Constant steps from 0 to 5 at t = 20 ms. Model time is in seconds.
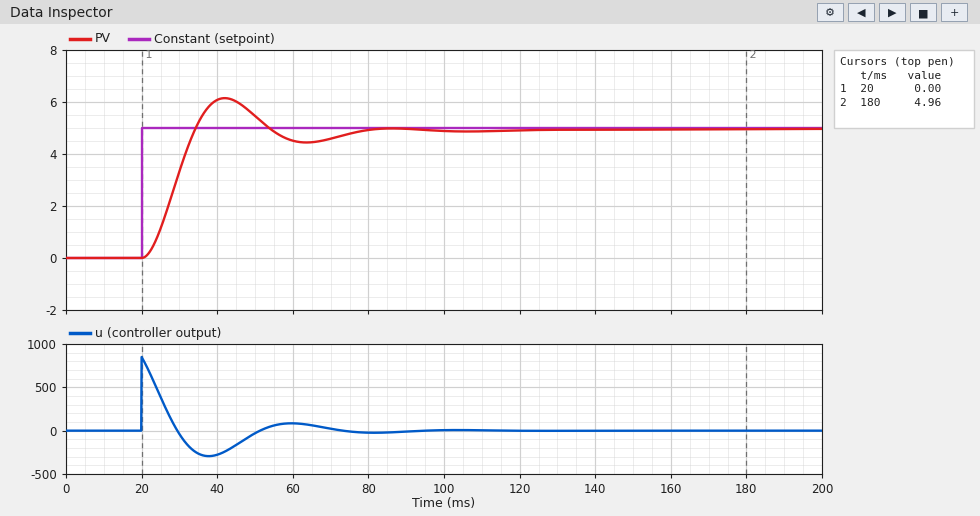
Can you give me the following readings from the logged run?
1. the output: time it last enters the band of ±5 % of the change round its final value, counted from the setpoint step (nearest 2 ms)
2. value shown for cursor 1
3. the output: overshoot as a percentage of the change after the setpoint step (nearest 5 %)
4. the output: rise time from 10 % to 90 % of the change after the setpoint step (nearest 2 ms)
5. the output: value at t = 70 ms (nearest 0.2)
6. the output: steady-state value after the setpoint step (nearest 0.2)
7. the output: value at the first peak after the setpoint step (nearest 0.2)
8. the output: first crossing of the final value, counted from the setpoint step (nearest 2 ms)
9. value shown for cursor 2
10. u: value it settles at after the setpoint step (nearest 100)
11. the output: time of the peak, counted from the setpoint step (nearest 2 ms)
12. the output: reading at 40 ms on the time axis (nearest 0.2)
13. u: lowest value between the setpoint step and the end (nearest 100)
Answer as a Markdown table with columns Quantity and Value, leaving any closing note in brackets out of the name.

| Quantity | Value |
|---|---|
| the output: time it last enters the band of ±5 % of the change round its final value, counted from the setpoint step | 54 ms |
| value shown for cursor 1 | 0.00 |
| the output: overshoot as a percentage of the change after the setpoint step | 25 % |
| the output: rise time from 10 % to 90 % of the change after the setpoint step | 10 ms |
| the output: value at t = 70 ms | 4.6 |
| the output: steady-state value after the setpoint step | 5.0 |
| the output: value at the first peak after the setpoint step | 6.2 |
| the output: first crossing of the final value, counted from the setpoint step | 14 ms |
| value shown for cursor 2 | 4.96 |
| u: value it settles at after the setpoint step | 0 |
| the output: time of the peak, counted from the setpoint step | 22 ms |
| the output: reading at 40 ms on the time axis | 6.0 |
| u: lowest value between the setpoint step and the end | -300 |
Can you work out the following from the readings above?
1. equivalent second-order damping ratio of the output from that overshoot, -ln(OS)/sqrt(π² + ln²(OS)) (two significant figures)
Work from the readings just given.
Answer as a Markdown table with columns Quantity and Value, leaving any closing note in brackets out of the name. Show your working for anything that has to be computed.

| Quantity | Value |
|---|---|
| equivalent second-order damping ratio of the output from that overshoot, -ln(OS)/sqrt(π² + ln²(OS)) | ln(0.25) = -1.386; 1.386 / sqrt(9.870 + 1.922) = 0.40 |
